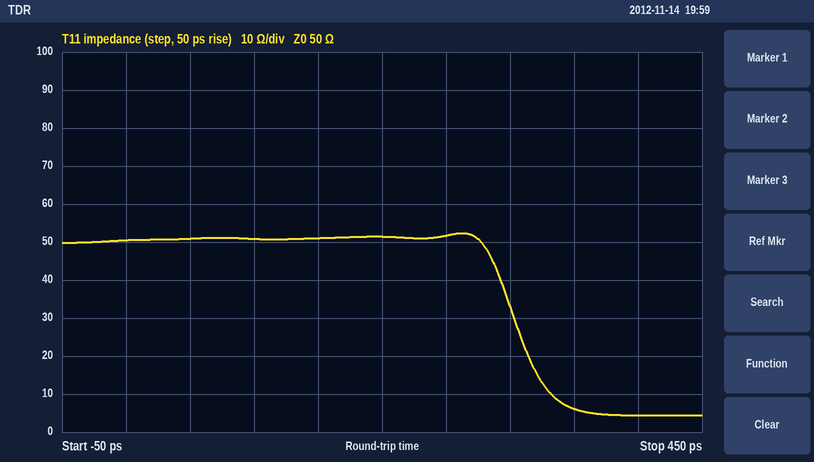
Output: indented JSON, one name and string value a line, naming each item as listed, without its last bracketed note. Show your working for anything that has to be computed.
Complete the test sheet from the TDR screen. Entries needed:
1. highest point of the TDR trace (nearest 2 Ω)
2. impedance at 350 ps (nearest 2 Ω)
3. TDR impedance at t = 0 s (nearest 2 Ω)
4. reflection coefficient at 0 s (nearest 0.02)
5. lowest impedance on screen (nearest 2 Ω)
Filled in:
{
  "highest point of the TDR trace": "52 Ω",
  "impedance at 350 ps": "6 Ω",
  "TDR impedance at t = 0 s": "50 Ω",
  "reflection coefficient at 0 s": "(50 − 50)/(50 + 50) ≈ 0.00",
  "lowest impedance on screen": "4 Ω"
}
